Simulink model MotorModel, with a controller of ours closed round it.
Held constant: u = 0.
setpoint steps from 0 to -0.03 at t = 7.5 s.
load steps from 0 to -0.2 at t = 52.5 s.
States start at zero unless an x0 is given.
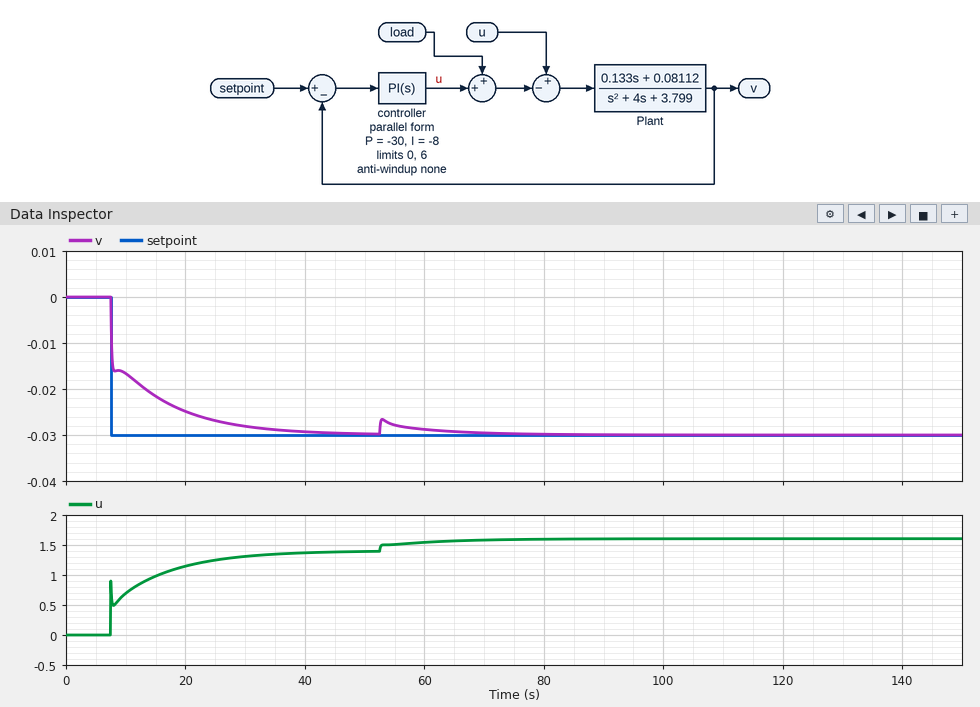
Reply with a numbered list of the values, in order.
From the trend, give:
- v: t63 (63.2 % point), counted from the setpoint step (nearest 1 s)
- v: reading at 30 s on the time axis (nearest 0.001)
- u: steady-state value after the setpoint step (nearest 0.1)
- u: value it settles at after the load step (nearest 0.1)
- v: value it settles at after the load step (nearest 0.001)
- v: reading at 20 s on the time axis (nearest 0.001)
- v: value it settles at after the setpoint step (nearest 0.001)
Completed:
1. 5 s
2. -0.028
3. 1.4
4. 1.6
5. -0.030
6. -0.025
7. -0.030
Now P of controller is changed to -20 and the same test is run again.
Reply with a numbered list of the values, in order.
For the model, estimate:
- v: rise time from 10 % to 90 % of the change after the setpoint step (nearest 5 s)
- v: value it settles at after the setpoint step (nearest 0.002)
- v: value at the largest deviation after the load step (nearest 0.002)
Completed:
1. 15 s
2. -0.030
3. -0.026
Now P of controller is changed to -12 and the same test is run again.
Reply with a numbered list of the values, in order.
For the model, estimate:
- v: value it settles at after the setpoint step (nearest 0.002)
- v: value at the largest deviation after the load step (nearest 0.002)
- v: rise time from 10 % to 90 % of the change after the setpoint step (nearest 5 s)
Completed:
1. -0.030
2. -0.026
3. 15 s
